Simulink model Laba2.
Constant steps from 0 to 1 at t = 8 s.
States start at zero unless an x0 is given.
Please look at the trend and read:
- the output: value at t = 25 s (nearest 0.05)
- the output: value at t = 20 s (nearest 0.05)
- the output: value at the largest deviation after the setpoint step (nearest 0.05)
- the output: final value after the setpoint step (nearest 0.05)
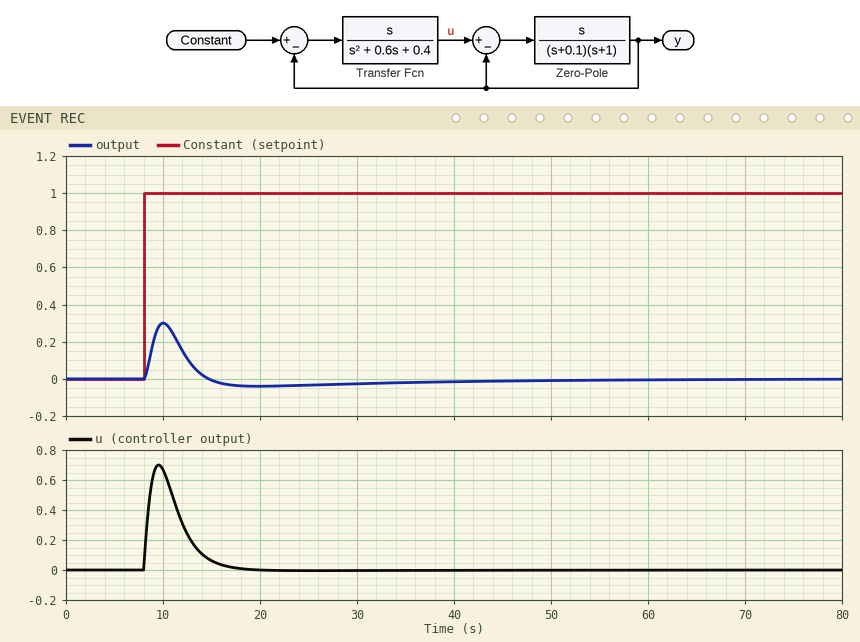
-0.05
-0.05
0.30
0.00
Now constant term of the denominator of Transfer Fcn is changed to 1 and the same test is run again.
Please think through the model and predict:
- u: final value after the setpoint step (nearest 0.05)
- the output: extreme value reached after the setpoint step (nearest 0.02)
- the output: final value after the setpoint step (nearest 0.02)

0.00
0.24
0.00
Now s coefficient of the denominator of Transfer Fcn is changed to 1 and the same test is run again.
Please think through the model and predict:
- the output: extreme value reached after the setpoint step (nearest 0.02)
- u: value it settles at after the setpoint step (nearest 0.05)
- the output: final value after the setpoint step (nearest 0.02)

0.24
0.00
0.00
